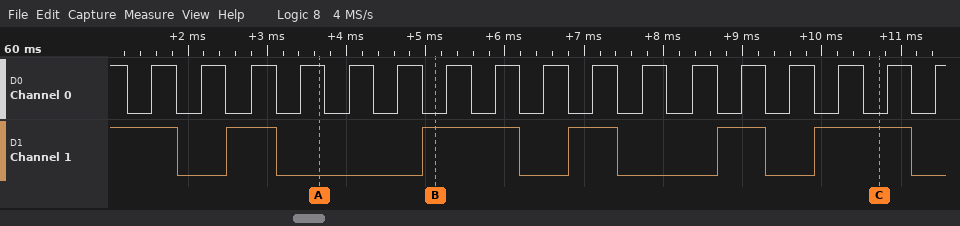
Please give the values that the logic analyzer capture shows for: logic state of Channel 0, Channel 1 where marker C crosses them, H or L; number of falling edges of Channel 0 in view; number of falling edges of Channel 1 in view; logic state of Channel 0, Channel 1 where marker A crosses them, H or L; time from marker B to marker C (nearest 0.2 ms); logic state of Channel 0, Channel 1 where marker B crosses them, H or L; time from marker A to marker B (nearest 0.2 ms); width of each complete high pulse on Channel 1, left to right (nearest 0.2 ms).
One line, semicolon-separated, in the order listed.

Channel 0=L, Channel 1=H; 17; 6; Channel 0=H, Channel 1=L; 5.6 ms; Channel 0=L, Channel 1=H; 1.4 ms; 0.6 ms, 1.2 ms, 0.6 ms, 0.6 ms, 1.2 ms
